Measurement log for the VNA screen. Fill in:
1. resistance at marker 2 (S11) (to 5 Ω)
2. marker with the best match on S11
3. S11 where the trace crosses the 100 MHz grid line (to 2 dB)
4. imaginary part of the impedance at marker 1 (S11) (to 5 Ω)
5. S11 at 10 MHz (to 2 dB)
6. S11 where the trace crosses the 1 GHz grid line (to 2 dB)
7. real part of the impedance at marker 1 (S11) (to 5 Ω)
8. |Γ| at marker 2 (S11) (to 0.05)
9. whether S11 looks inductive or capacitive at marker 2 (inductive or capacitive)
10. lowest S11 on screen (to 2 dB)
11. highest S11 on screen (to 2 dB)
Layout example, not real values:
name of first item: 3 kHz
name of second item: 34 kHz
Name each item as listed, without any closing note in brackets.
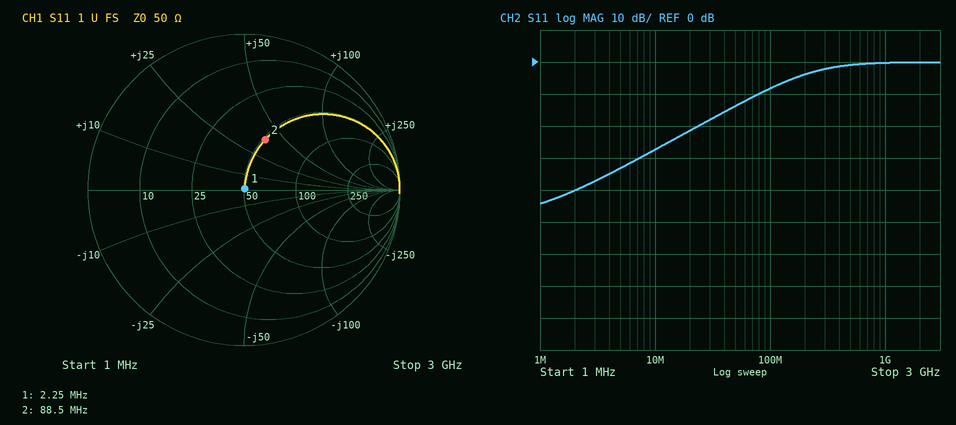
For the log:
resistance at marker 2 (S11): 50 Ω
marker with the best match on S11: marker 1
S11 where the trace crosses the 100 MHz grid line: -8 dB
imaginary part of the impedance at marker 1 (S11): 0 Ω
S11 at 10 MHz: -28 dB
S11 where the trace crosses the 1 GHz grid line: 0 dB
real part of the impedance at marker 1 (S11): 50 Ω
|Γ| at marker 2 (S11): 0.35
whether S11 looks inductive or capacitive at marker 2: inductive
lowest S11 on screen: -44 dB
highest S11 on screen: 0 dB
